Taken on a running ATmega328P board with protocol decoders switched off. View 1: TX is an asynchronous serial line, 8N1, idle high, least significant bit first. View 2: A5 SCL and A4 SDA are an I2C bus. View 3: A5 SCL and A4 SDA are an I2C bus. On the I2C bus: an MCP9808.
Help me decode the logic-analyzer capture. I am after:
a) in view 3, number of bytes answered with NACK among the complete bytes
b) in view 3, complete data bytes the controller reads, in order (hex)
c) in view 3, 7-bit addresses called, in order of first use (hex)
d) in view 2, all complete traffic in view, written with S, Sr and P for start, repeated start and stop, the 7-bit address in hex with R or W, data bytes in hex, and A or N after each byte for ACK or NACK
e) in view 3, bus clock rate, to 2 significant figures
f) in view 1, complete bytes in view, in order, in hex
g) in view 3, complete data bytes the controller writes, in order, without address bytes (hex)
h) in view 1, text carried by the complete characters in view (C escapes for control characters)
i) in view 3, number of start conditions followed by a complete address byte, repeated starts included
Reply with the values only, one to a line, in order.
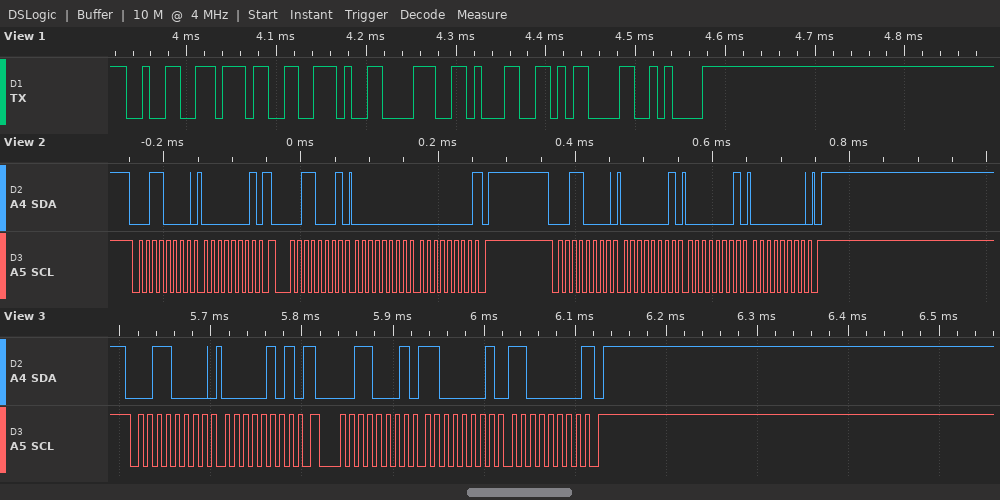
1
C1 C0
0x18
S 18W A 01 A Sr 18R A 00 A 00 N P S 18W A 01 A 01 A 00 A P
100 kHz
32 37 2E 38 31 0D 0A
05
"27.81\r\n"
2
